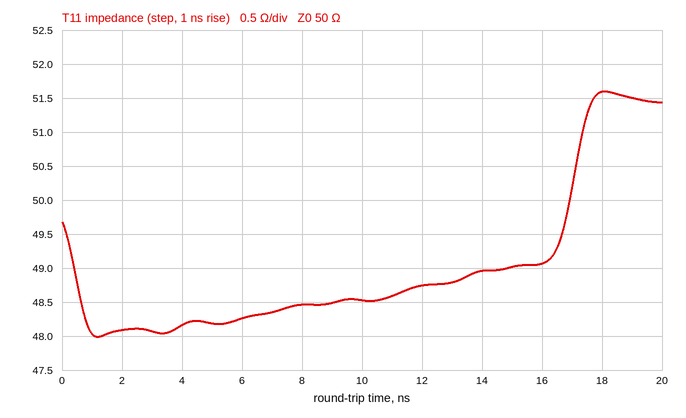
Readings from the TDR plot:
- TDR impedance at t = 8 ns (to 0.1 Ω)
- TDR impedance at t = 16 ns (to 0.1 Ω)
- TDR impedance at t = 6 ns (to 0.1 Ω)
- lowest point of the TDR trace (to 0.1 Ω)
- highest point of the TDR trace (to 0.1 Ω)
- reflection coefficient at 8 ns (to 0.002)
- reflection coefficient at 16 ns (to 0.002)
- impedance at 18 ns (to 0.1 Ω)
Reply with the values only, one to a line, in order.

48.5 Ω
49.1 Ω
48.3 Ω
48.0 Ω
51.6 Ω
-0.016
-0.010
51.6 Ω
